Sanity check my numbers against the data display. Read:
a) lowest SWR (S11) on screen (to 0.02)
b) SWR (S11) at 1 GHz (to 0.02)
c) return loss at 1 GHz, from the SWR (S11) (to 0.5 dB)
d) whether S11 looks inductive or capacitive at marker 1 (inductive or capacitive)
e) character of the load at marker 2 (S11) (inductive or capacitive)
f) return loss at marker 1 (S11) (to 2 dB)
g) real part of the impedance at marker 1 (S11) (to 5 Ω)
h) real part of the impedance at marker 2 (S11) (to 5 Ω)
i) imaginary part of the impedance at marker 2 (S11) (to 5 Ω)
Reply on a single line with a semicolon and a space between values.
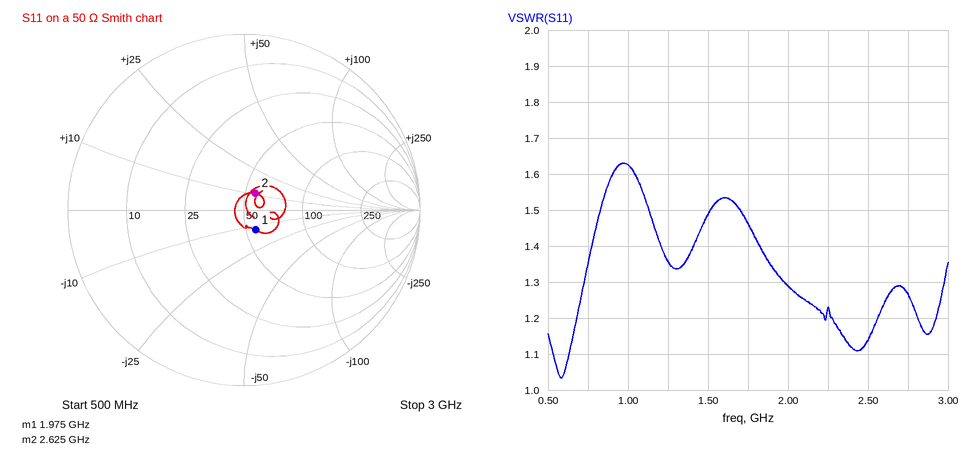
1.04; 1.62; 12.5 dB; capacitive; inductive; 18 dB; 55 Ω; 55 Ω; +10 Ω
